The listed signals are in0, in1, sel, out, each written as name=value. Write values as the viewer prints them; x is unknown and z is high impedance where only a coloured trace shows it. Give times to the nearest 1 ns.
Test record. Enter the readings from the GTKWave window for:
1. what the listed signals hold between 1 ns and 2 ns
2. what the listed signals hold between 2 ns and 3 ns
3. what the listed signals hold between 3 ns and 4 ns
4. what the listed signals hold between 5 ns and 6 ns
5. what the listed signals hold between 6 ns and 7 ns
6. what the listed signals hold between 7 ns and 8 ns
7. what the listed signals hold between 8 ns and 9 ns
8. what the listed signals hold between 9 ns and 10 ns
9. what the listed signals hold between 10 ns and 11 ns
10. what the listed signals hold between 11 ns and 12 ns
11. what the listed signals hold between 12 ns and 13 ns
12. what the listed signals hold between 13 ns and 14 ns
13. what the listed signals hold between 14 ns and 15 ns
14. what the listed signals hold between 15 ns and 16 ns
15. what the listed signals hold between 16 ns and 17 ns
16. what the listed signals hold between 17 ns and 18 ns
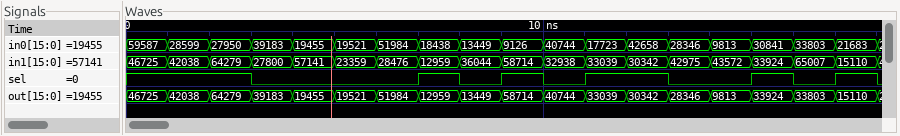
in0=28599, in1=42038, sel=1, out=42038
in0=27950, in1=64279, sel=1, out=64279
in0=39183, in1=27800, sel=0, out=39183
in0=19521, in1=23359, sel=0, out=19521
in0=51984, in1=28476, sel=0, out=51984
in0=18438, in1=12959, sel=1, out=12959
in0=13449, in1=36044, sel=0, out=13449
in0=9126, in1=58714, sel=1, out=58714
in0=40744, in1=32938, sel=0, out=40744
in0=17723, in1=33039, sel=1, out=33039
in0=42658, in1=30342, sel=1, out=30342
in0=28346, in1=42975, sel=0, out=28346
in0=9813, in1=43572, sel=0, out=9813
in0=30841, in1=33924, sel=1, out=33924
in0=33803, in1=65007, sel=0, out=33803
in0=21683, in1=15110, sel=1, out=15110
